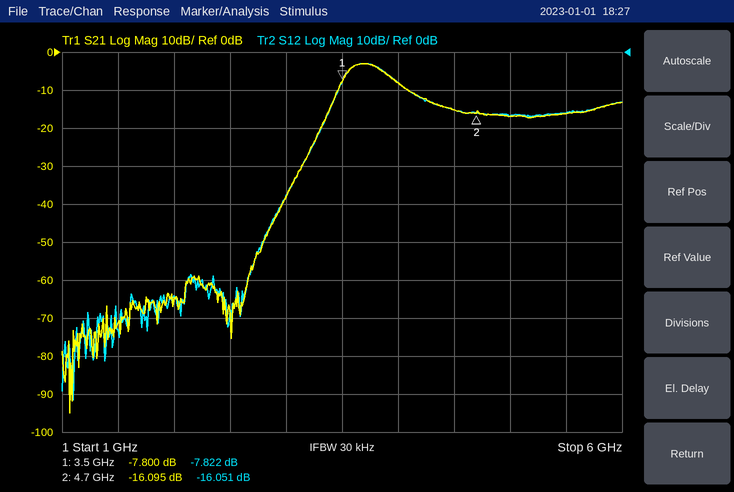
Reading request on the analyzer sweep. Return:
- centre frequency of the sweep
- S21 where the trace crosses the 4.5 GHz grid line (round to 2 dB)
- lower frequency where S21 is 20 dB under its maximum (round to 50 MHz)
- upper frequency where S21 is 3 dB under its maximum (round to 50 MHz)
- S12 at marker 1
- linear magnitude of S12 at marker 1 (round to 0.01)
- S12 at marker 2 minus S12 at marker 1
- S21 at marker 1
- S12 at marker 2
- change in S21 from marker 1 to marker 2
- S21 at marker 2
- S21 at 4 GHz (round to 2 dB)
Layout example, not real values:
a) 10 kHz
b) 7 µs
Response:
a) 3.5 GHz
b) -16 dB
c) 3.25 GHz
d) 3.90 GHz
e) -7.822 dB
f) 0.41
g) -8.229 dB
h) -7.800 dB
i) -16.051 dB
j) -8.295 dB
k) -16.095 dB
l) -8 dB
